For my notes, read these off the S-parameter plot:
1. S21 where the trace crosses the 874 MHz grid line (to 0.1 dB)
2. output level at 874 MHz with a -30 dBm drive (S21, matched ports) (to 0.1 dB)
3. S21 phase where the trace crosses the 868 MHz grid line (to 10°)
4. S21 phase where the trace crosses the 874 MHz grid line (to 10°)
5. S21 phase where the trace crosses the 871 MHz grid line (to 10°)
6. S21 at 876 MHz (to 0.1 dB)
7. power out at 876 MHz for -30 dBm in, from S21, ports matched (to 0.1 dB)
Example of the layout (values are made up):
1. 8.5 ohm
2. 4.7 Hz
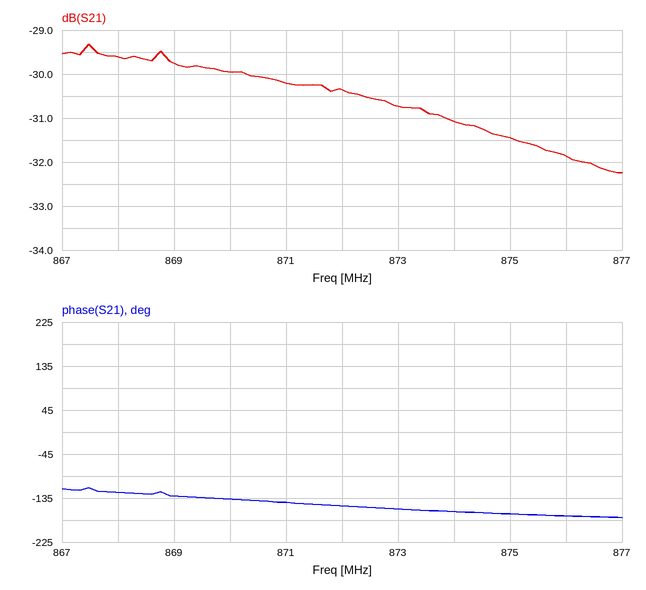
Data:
1. -31.1 dB
2. -61.1 dBm
3. -120°
4. -160°
5. -140°
6. -31.9 dB
7. -61.9 dBm
